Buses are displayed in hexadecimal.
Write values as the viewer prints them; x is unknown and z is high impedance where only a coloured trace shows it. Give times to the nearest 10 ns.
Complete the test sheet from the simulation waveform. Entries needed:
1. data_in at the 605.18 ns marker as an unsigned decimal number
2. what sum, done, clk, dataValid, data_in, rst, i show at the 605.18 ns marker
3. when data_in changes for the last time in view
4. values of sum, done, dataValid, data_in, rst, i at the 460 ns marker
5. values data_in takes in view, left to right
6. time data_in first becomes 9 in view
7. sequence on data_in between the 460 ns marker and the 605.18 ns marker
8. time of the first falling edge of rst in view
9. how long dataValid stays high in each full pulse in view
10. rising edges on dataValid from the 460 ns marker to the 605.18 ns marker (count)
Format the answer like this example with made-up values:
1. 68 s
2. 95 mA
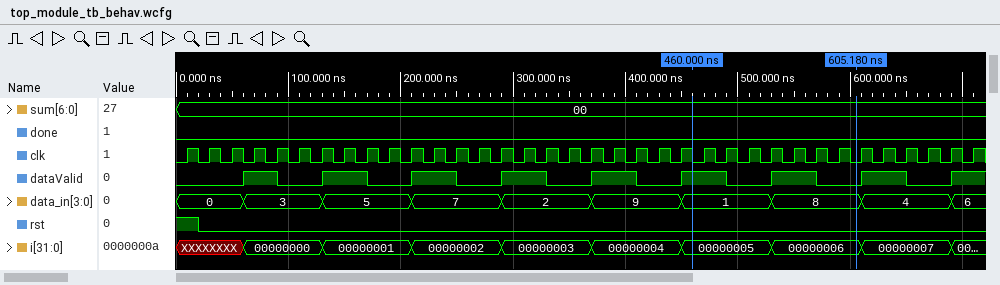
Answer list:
1. 8
2. sum=00, done=0, clk=0, dataValid=0, data_in=8, rst=0, i=00000006
3. 690 ns
4. sum=00, done=0, dataValid=1, data_in=1, rst=0, i=00000005
5. 0, 3, 5, 7, 2, 9, 1, 8, 4, 6
6. 370 ns
7. 1, 8
8. 20 ns
9. 30 ns, 40 ns, 40 ns, 40 ns, 40 ns, 40 ns, 40 ns, 40 ns
10. 1
